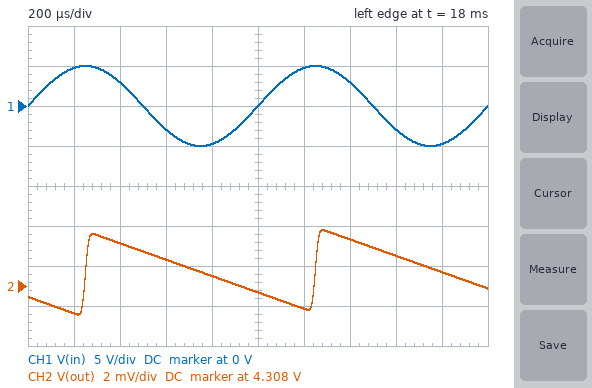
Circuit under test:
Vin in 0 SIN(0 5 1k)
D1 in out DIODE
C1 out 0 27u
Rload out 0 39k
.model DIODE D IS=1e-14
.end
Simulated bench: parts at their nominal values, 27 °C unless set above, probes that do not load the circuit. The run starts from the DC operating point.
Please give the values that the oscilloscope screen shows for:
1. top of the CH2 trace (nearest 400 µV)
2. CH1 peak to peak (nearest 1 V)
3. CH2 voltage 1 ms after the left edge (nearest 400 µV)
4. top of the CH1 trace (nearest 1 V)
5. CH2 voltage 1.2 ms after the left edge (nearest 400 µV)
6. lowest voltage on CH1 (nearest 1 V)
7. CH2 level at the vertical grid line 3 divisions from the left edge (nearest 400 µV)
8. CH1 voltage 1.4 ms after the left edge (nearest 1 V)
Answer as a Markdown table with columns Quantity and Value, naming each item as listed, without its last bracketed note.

| Quantity | Value |
|---|---|
| top of the CH2 trace | 4.3108 V |
| CH1 peak to peak | 10 V |
| CH2 voltage 1 ms after the left edge | 4.3076 V |
| top of the CH1 trace | 5 V |
| CH2 voltage 1.2 ms after the left edge | 4.3068 V |
| lowest voltage on CH1 | -5 V |
| CH2 level at the vertical grid line 3 divisions from the left edge | 4.3092 V |
| CH1 voltage 1.4 ms after the left edge | 3 V |
